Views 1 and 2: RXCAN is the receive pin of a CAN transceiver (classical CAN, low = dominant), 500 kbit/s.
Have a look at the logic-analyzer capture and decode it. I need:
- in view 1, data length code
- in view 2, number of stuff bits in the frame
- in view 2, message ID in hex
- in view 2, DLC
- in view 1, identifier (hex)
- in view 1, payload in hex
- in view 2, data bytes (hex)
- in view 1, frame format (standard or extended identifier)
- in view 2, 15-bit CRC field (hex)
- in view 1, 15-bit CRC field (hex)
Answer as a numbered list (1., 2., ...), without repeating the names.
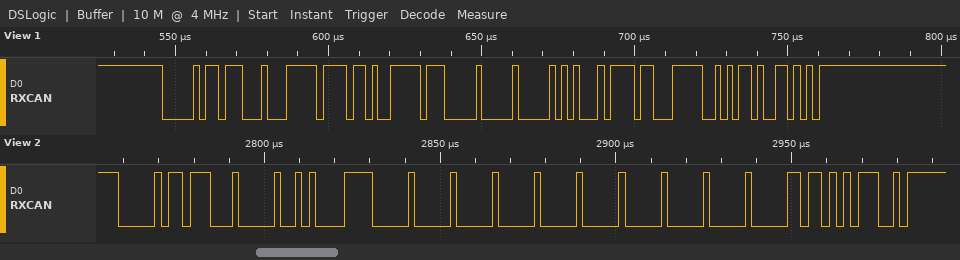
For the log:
1. 8
2. 12
3. 0x037
4. 8
5. 0x037
6. FF B4 FF 00 00 A2 F6 3E
7. 0A 1E 00 00 00 00 00 00
8. standard
9. 0x2D5C
10. 0x569A
